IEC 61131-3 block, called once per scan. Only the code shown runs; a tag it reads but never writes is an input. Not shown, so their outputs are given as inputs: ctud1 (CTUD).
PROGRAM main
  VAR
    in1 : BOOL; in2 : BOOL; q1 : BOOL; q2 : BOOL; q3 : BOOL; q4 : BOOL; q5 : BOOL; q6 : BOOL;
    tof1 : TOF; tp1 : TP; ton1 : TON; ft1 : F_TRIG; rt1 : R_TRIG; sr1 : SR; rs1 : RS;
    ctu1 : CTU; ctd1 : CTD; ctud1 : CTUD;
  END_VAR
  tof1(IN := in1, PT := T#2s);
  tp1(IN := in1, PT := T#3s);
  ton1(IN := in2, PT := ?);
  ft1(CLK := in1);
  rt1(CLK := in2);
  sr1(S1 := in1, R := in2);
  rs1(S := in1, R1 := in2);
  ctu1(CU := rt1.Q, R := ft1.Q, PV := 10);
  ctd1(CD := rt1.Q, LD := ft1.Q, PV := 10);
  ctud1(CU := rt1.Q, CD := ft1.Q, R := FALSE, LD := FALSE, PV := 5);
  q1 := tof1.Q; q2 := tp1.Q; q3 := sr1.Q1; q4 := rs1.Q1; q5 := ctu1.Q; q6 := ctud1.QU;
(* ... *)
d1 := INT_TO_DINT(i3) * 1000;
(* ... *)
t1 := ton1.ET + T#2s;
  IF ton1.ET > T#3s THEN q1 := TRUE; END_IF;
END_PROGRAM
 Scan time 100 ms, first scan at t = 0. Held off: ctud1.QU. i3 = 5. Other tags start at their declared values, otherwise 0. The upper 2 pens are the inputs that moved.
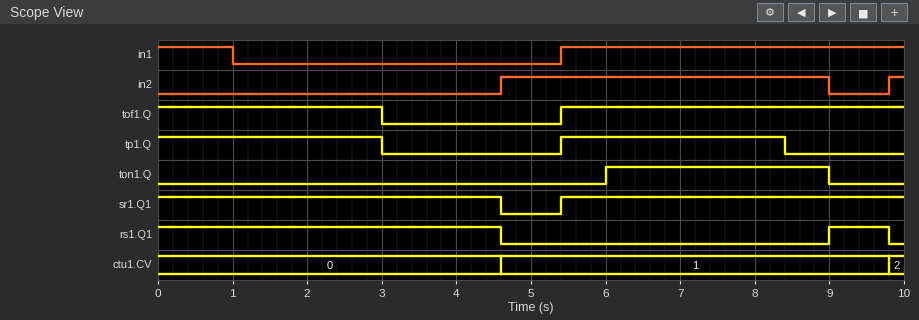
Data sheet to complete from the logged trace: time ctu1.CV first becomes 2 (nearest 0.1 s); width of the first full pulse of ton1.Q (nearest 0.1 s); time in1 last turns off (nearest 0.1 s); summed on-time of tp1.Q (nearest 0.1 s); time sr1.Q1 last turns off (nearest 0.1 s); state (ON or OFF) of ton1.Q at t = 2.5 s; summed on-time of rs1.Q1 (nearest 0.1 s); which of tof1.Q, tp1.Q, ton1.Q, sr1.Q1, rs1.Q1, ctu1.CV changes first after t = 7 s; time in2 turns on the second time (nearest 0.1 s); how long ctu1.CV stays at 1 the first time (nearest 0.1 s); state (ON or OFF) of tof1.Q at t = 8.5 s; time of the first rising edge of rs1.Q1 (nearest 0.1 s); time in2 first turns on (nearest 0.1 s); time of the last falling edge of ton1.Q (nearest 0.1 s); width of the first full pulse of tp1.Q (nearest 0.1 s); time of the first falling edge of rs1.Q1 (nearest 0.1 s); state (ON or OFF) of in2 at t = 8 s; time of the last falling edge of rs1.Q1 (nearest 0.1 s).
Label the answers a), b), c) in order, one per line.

a) 9.8 s
b) 3.0 s
c) 1.0 s
d) 6.0 s
e) 4.6 s
f) OFF
g) 5.4 s
h) tp1.Q
i) 9.8 s
j) 5.2 s
k) ON
l) 9.0 s
m) 4.6 s
n) 9.0 s
o) 3.0 s
p) 4.6 s
q) ON
r) 9.8 s
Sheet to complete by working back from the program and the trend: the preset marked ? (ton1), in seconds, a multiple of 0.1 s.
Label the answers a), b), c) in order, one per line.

a) 1.4 s
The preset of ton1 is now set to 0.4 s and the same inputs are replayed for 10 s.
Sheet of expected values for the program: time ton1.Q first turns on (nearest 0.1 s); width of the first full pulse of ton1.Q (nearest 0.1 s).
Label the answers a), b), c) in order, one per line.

a) 5.0 s
b) 4.0 s
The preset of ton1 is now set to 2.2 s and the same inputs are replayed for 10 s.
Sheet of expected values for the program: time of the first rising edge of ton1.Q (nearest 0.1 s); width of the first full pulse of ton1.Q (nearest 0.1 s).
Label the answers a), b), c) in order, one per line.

a) 6.8 s
b) 2.2 s
